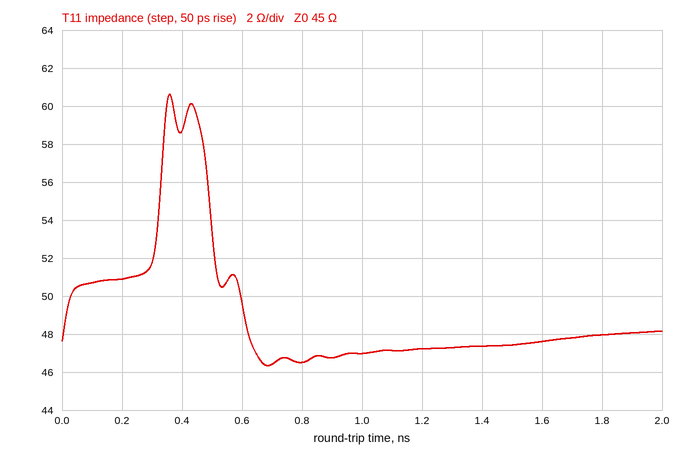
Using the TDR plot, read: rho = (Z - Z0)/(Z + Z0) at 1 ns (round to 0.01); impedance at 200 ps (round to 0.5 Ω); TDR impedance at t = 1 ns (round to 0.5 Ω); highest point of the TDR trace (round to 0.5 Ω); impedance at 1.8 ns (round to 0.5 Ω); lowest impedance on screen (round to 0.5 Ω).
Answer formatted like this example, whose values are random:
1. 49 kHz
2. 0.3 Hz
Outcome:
1. +0.02
2. 51.0 Ω
3. 47.0 Ω
4. 60.5 Ω
5. 48.0 Ω
6. 46.5 Ω
